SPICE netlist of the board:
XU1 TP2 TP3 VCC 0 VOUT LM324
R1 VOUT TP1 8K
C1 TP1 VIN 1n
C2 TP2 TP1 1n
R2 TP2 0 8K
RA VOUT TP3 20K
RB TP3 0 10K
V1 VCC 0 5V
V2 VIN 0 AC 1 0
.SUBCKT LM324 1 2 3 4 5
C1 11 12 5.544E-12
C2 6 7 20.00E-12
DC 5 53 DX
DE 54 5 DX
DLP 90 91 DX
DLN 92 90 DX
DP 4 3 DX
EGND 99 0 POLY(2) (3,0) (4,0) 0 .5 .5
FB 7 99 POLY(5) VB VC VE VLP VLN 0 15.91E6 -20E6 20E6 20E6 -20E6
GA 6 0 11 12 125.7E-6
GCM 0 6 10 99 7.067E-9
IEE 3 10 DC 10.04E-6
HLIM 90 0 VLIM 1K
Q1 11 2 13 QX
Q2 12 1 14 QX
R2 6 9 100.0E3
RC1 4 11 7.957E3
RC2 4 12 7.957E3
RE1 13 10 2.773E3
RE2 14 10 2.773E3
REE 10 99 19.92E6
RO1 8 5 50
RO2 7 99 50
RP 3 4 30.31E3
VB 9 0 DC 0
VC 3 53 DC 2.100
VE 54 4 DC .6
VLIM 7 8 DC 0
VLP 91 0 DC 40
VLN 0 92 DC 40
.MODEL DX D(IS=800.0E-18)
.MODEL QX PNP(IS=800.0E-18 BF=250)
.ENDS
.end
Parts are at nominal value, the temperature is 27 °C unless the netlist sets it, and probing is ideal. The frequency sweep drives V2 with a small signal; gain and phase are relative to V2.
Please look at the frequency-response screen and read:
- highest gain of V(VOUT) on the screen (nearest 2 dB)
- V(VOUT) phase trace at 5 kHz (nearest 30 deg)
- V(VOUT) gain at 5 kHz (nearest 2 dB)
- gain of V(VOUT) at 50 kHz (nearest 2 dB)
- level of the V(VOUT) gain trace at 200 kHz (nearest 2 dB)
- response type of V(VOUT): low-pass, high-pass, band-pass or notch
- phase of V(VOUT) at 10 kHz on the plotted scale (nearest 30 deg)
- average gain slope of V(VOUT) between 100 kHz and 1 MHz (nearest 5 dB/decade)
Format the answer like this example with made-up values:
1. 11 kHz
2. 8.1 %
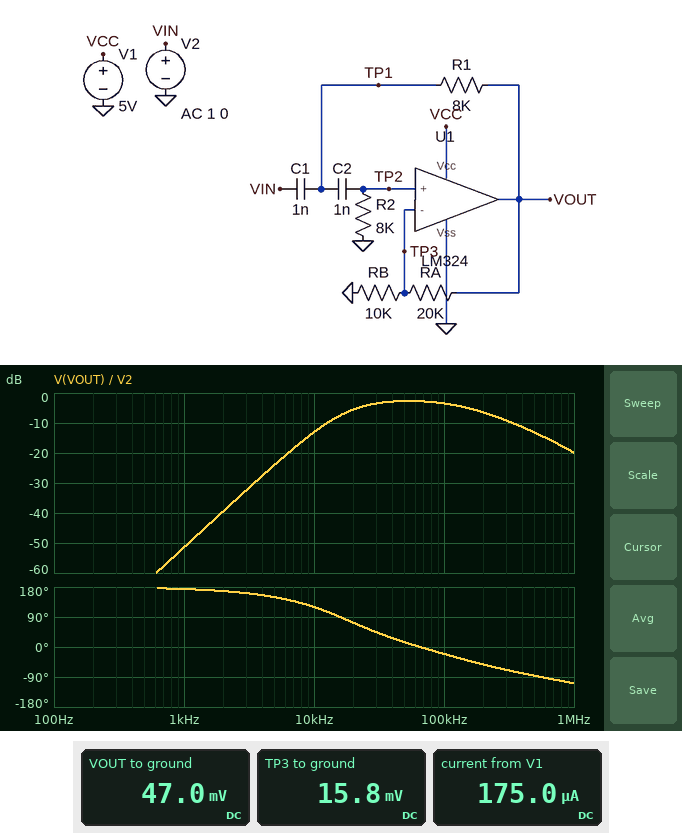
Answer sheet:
1. -2 dB
2. 150 deg
3. -24 dB
4. -2 dB
5. -6 dB
6. band-pass
7. 120 deg
8. -15 dB/decade
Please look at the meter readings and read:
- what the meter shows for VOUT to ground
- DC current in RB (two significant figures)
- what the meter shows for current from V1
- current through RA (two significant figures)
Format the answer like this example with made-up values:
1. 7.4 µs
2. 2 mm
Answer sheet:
1. 47.0 mV
2. 1.6 µA
3. 175.0 µA
4. 1.6 µA
